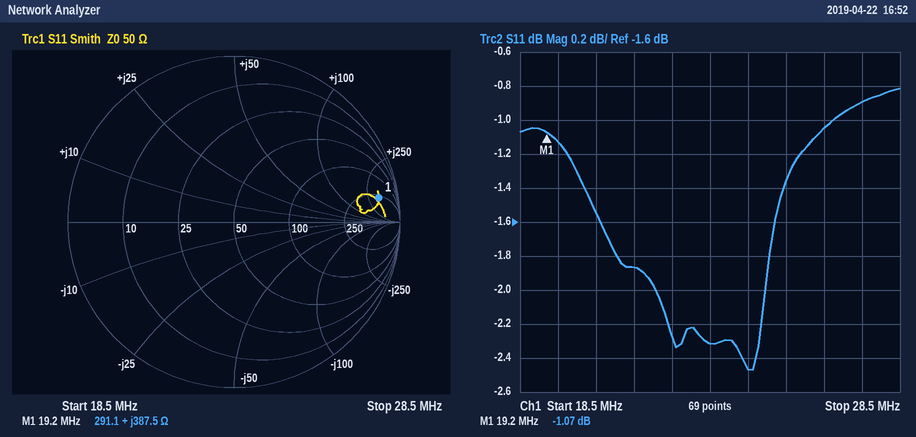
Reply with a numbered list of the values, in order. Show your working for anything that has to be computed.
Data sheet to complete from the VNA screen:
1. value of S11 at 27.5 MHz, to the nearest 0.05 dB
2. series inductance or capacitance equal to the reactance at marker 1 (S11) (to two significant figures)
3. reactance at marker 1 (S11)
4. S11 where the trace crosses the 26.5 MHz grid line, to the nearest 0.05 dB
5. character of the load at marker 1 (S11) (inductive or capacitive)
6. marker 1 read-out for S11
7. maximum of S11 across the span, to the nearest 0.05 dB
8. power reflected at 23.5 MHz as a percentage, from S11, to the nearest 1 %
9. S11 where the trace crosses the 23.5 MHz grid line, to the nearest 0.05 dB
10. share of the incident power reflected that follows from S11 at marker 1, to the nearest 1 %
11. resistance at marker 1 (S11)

1. -0.90 dB
2. L = 387.5 Ω/(2π × 19.2 MHz) ≈ 3.2 µH
3. +387.5 Ω
4. -1.05 dB
5. inductive
6. -1.07 dB
7. -0.80 dB
8. 10^(-2.3/10) ≈ 59 %
9. -2.30 dB
10. 10^(-1.07/10) ≈ 78 %
11. 291.1 Ω
